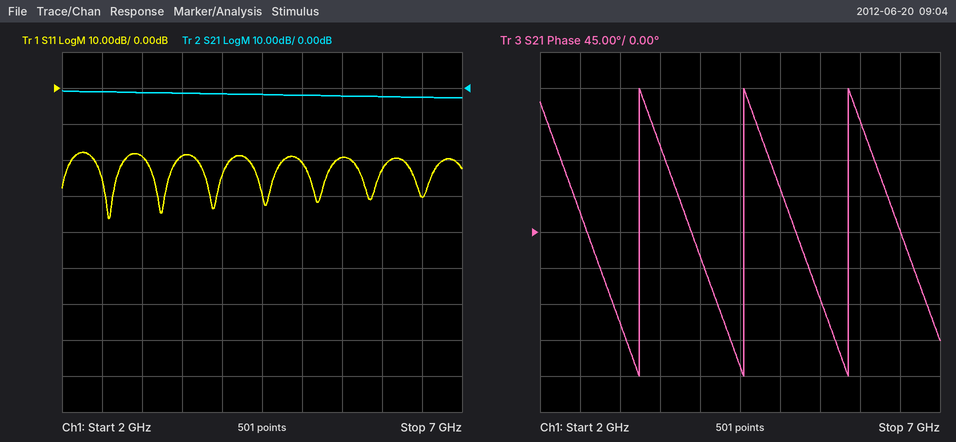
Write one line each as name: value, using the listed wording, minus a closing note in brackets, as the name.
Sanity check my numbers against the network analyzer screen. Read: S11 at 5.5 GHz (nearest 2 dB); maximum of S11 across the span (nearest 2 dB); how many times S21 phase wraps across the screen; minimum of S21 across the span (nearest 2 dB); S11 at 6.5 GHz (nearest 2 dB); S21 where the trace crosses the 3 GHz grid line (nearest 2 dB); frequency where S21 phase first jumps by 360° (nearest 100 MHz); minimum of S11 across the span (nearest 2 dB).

S11 at 5.5 GHz: -20 dB
maximum of S11 across the span: -18 dB
how many times S21 phase wraps across the screen: 3
minimum of S21 across the span: -2 dB
S11 at 6.5 GHz: -30 dB
S21 where the trace crosses the 3 GHz grid line: -2 dB
frequency where S21 phase first jumps by 360°: 3.2 GHz
minimum of S11 across the span: -36 dB
